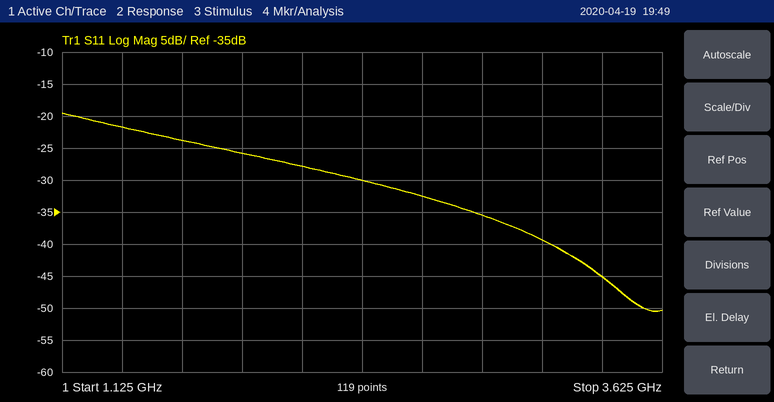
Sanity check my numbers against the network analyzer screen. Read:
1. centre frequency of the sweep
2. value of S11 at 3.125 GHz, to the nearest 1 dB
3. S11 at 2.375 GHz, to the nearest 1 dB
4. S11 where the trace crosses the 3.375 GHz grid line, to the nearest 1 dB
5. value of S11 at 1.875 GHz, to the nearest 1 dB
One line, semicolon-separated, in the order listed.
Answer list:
2.375 GHz; -39 dB; -30 dB; -45 dB; -26 dB
